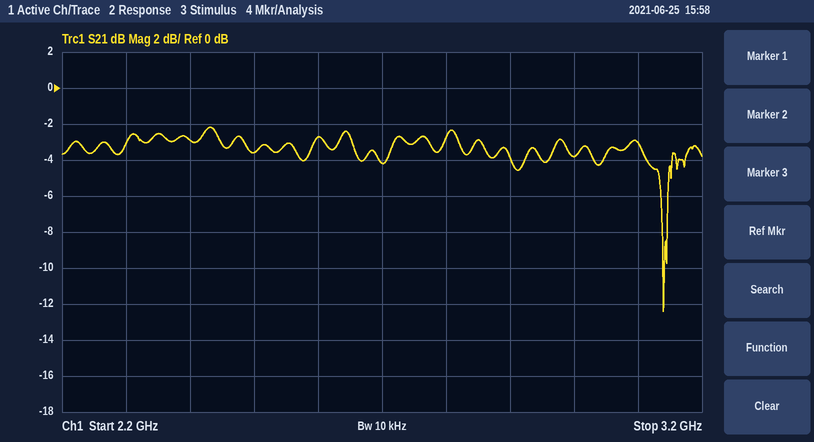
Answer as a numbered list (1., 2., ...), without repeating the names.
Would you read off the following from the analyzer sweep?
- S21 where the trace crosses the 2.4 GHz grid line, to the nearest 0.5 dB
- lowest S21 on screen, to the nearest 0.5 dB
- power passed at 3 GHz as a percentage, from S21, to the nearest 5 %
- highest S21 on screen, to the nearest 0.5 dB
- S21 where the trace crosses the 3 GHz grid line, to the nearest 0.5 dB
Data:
1. -3.0 dB
2. -12.5 dB
3. 40 %
4. -2.0 dB
5. -4.0 dB
